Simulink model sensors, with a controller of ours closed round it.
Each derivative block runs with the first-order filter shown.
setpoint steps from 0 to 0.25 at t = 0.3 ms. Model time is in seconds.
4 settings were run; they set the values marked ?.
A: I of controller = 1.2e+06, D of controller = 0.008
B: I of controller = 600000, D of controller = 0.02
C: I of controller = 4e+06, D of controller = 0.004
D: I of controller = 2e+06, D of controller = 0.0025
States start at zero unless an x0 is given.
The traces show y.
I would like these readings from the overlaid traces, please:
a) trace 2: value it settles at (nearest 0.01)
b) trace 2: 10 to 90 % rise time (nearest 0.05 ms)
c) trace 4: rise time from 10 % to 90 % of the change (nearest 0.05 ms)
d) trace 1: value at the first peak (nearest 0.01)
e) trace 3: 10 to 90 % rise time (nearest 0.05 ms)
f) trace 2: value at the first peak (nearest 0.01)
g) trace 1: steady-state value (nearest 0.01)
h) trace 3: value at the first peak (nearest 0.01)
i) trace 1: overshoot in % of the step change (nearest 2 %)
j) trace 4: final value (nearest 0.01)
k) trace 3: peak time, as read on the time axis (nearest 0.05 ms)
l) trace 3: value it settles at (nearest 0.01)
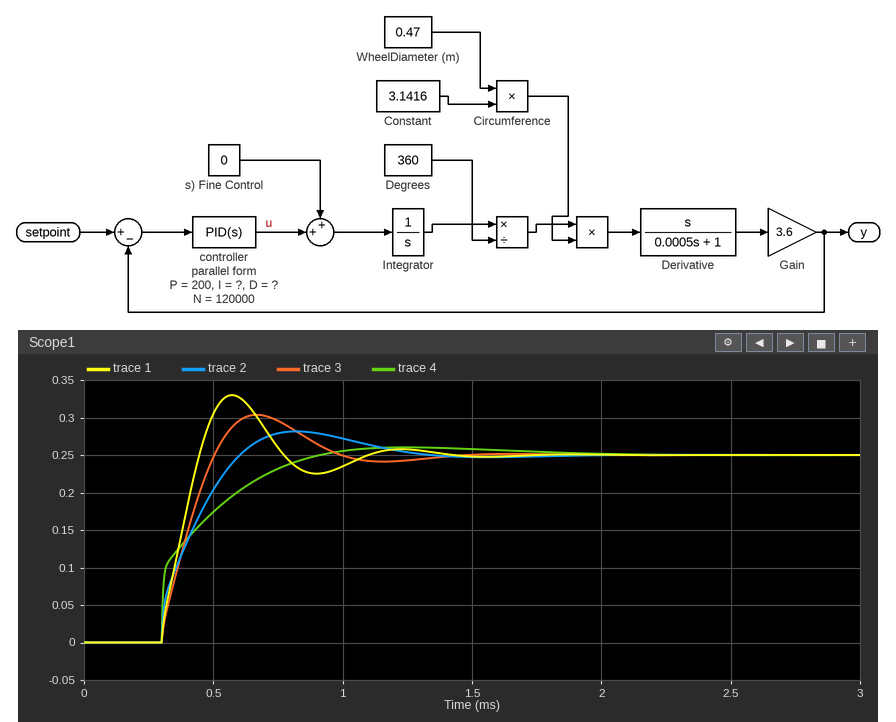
0.25
0.25 ms
0.40 ms
0.33
0.15 ms
0.28
0.25
0.30
32 %
0.25
0.65 ms
0.25
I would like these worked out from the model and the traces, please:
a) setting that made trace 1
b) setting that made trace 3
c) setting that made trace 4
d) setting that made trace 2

C
D
B
A
